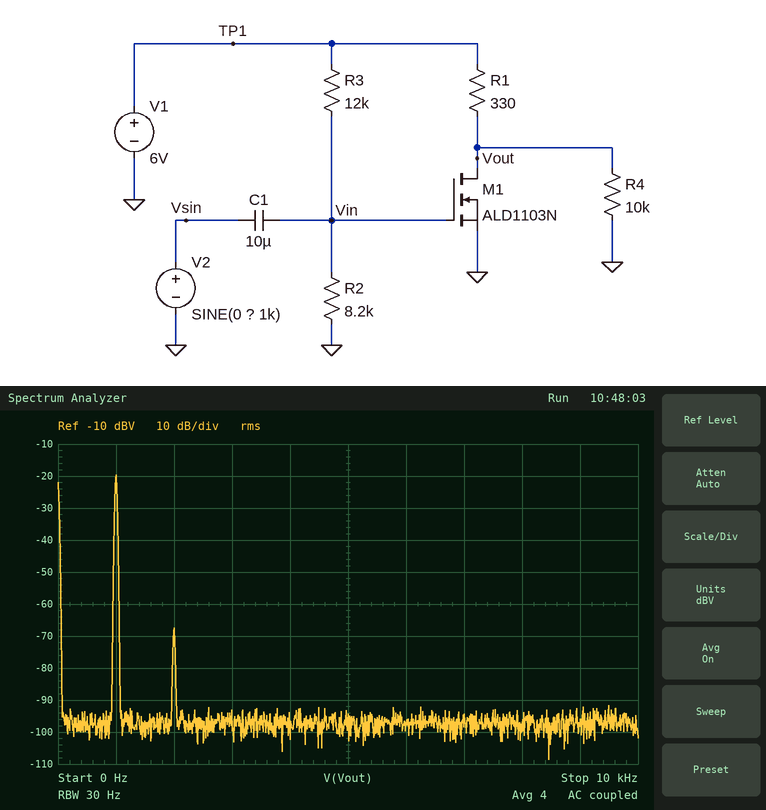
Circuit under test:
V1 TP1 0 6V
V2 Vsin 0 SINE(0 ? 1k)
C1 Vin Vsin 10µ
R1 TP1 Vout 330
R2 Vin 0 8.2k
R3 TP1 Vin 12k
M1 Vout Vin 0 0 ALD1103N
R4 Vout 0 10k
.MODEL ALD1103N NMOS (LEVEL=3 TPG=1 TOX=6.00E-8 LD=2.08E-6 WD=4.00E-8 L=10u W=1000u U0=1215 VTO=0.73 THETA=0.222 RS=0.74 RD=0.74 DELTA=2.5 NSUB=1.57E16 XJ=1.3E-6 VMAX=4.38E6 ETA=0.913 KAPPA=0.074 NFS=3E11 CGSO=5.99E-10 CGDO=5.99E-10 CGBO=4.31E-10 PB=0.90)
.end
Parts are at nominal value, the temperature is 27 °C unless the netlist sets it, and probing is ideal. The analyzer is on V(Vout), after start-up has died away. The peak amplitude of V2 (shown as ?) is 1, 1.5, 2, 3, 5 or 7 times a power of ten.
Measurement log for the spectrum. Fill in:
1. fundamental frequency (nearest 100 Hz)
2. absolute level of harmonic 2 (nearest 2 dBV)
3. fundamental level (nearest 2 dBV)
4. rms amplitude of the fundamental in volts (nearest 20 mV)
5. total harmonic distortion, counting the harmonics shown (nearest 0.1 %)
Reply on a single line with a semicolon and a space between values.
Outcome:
1.0 kHz; -68 dBV; -20 dBV; 100 mV; 0.4 %
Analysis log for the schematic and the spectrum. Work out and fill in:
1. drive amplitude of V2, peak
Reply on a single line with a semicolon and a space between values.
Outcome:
50 mV
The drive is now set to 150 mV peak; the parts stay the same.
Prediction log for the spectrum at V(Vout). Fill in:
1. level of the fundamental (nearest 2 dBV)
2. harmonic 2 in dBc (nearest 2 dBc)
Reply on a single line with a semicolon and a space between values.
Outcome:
-10 dBV; -38 dBc
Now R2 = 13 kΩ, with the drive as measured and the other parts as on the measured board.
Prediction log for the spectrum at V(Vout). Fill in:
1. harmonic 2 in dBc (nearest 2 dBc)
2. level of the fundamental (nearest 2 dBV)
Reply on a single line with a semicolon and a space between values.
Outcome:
-30 dBc; -32 dBV
